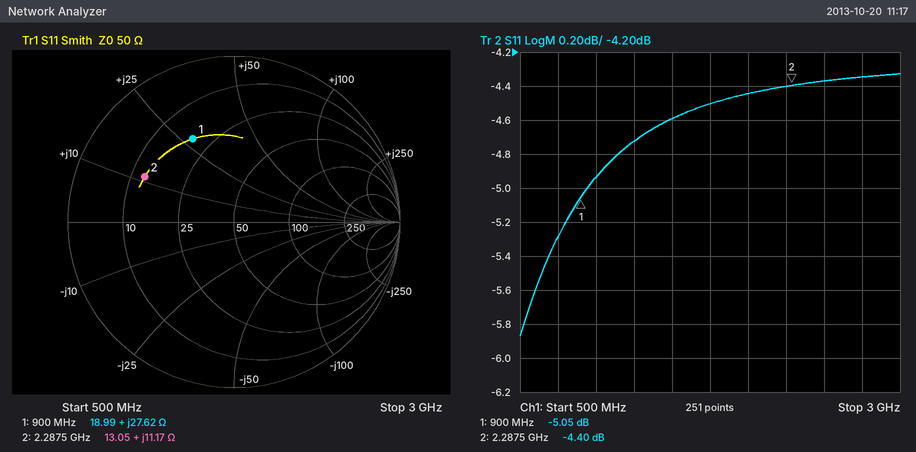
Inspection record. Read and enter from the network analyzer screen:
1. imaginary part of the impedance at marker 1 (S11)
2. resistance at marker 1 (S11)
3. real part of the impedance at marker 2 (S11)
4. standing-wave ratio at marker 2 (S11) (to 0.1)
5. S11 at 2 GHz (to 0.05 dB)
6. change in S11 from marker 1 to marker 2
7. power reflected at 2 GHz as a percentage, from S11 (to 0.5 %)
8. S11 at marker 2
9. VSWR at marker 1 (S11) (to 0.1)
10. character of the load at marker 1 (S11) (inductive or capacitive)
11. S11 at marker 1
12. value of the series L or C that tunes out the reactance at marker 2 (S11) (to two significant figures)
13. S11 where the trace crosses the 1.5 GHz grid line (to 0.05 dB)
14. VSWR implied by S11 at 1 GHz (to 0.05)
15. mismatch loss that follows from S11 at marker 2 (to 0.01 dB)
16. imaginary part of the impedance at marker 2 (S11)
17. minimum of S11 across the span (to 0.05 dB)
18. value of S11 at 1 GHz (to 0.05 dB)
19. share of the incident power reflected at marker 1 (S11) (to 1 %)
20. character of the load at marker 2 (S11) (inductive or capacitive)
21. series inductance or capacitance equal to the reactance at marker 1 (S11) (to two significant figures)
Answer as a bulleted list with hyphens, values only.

- +27.62 Ω
- 18.99 Ω
- 13.05 Ω
- 4.0
- -4.45 dB
- 0.65 dB
- 36.0 %
- -4.40 dB
- 3.5
- inductive
- -5.05 dB
- 6.2 pF
- -4.60 dB
- 3.60
- 1.96 dB
- +11.17 Ω
- -5.85 dB
- -4.95 dB
- 31 %
- inductive
- 4.9 nH
